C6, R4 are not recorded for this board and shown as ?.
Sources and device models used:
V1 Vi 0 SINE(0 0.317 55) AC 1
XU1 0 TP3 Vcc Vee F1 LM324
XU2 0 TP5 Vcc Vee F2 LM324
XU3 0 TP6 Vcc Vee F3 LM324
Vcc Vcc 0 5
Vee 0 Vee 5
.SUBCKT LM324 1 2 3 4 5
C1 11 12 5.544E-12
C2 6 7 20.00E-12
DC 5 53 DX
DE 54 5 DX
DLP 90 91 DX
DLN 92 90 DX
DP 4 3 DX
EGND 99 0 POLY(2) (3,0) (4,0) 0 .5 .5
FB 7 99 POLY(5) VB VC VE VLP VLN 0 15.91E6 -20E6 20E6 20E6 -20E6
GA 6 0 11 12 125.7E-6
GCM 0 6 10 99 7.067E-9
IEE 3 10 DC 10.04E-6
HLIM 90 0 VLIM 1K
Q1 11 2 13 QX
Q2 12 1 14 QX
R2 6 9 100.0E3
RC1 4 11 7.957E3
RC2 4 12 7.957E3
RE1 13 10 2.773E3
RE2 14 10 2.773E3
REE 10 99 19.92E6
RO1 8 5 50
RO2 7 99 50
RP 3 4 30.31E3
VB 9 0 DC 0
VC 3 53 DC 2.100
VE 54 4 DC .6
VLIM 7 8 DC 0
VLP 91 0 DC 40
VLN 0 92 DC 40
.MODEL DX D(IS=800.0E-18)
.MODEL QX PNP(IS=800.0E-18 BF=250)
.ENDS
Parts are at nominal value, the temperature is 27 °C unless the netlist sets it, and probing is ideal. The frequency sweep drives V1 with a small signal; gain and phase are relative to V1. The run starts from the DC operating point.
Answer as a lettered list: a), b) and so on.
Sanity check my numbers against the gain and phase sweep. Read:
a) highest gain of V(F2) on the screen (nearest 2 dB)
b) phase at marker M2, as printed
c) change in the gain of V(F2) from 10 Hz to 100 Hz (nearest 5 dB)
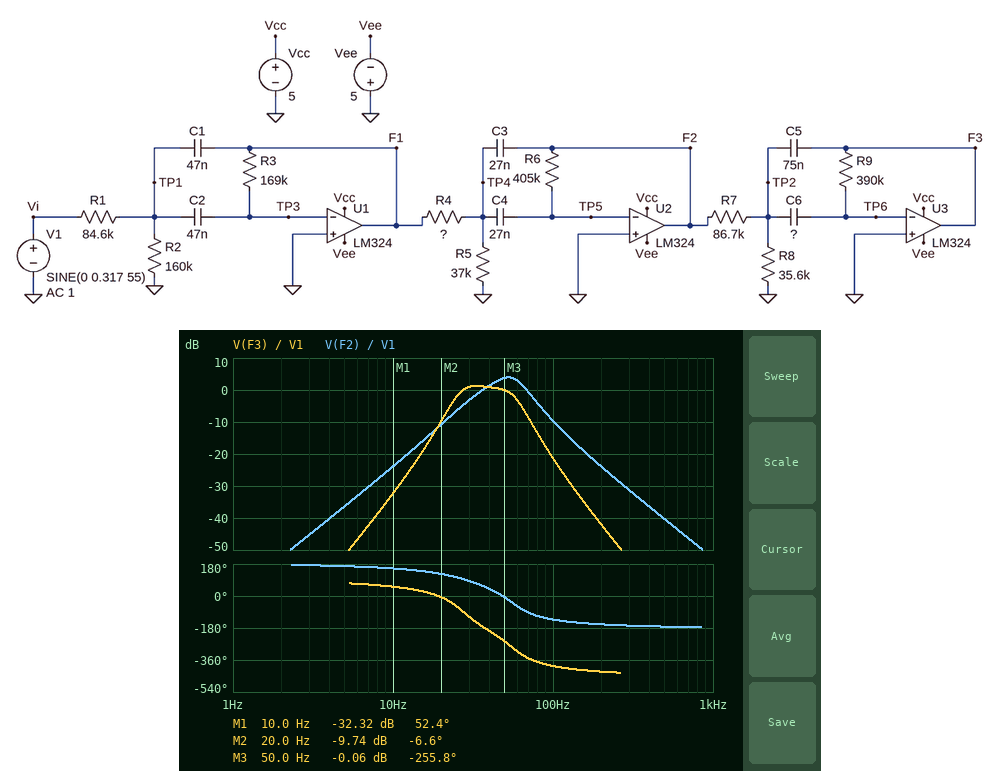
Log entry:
a) 4 dB
b) -6.6 deg
c) 15 dB
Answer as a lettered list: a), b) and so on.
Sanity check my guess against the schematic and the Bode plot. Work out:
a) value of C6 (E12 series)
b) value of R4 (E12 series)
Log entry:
a) 47 nF
b) 100 kΩ
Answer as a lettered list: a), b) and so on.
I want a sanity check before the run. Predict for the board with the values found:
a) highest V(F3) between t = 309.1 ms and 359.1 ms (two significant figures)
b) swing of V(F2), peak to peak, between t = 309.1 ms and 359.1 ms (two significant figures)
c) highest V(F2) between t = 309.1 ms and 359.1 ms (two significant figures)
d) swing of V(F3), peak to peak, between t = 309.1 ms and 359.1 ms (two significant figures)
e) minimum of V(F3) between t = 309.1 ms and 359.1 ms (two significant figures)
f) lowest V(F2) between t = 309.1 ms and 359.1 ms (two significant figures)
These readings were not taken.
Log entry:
a) 270 mV
b) 990 mV
c) 490 mV
d) 550 mV
e) -280 mV
f) -500 mV
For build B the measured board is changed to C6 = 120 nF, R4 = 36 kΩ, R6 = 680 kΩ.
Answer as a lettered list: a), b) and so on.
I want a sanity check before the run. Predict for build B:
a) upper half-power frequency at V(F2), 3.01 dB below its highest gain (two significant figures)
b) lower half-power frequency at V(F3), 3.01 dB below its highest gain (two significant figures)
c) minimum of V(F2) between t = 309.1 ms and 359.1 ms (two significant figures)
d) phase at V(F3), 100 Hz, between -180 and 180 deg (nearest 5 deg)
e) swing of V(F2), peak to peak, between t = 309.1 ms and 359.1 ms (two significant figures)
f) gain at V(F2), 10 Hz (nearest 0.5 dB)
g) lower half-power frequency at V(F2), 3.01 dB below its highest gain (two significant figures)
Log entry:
a) 60 Hz
b) 34 Hz
c) -2.3 V
d) -45 deg
e) 4.5 V
f) -14.0 dB
g) 43 Hz
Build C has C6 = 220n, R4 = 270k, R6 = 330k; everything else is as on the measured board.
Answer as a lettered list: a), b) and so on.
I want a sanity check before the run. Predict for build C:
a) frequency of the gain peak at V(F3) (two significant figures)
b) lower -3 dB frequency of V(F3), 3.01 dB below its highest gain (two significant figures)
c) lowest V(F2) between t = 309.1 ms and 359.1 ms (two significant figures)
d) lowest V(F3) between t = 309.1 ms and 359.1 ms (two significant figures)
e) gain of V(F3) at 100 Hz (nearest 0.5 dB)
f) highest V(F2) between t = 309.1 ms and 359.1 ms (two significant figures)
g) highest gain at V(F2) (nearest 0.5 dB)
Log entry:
a) 42 Hz
b) 21 Hz
c) -160 mV
d) -77 mV
e) -30.5 dB
f) 140 mV
g) -6.5 dB
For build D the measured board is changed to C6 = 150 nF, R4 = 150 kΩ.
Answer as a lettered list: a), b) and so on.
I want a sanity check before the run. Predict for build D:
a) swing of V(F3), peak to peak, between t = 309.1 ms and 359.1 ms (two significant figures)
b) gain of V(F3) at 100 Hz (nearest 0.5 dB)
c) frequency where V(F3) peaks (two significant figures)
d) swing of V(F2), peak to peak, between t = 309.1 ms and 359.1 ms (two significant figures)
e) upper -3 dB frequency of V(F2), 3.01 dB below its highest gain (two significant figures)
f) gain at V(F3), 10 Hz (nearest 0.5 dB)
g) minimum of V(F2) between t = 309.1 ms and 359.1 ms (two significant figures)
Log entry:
a) 310 mV
b) -25.5 dB
c) 44 Hz
d) 660 mV
e) 63 Hz
f) -22.5 dB
g) -340 mV
